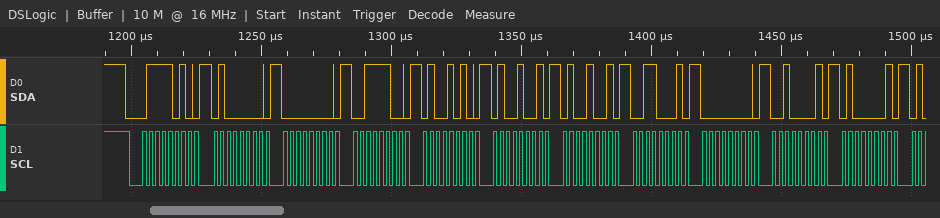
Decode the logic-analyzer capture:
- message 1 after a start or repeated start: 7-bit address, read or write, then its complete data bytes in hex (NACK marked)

0x3D write: 40 00 3C 4A 49 49 31 00 21 41
